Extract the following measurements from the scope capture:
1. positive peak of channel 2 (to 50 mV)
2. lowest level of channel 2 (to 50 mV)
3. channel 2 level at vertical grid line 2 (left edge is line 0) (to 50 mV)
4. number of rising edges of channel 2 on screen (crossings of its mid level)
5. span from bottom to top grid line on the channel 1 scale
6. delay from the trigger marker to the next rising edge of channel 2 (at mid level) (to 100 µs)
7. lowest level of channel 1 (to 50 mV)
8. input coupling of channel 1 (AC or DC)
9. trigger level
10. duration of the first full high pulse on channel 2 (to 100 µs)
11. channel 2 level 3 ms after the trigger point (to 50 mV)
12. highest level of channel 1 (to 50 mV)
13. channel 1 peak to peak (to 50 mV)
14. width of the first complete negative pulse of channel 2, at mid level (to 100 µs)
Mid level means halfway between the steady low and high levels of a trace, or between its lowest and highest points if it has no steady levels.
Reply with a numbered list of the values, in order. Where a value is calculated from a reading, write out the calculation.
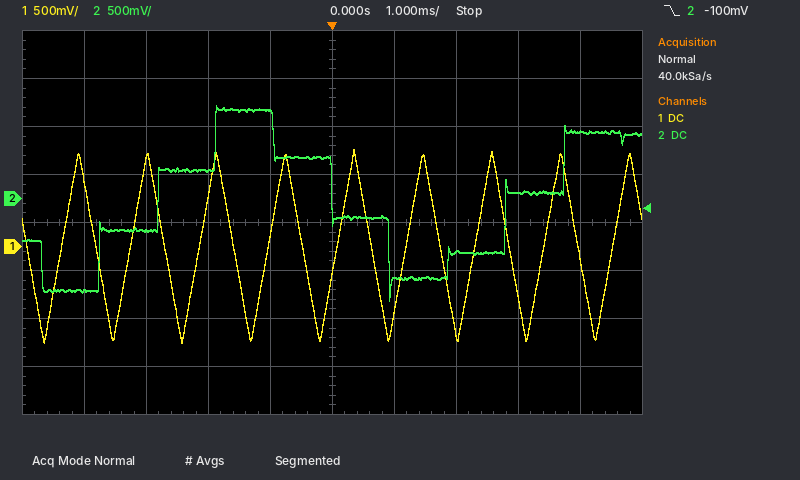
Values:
1. 950 mV
2. -1.05 V
3. -350 mV
4. 2
5. 4 V
6. 2.8 ms
7. -1.00 V
8. DC
9. -100 mV
10. 2.8 ms
11. 50 mV
12. 1.00 V
13. 1.00 V − (-1.00 V) = 2.00 V
14. 2.8 ms
